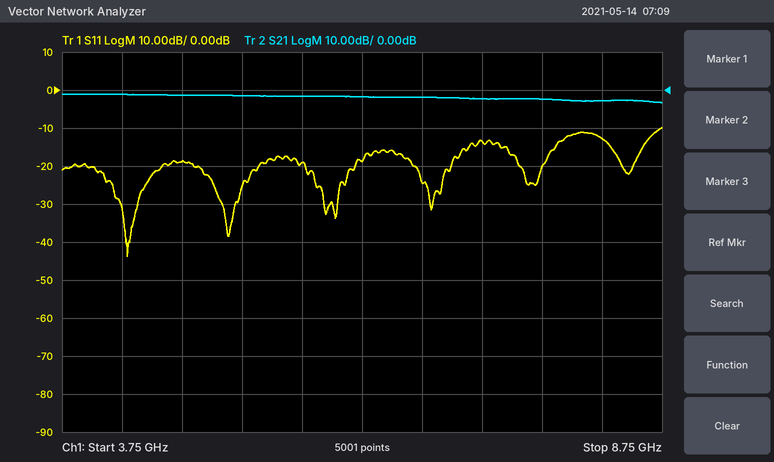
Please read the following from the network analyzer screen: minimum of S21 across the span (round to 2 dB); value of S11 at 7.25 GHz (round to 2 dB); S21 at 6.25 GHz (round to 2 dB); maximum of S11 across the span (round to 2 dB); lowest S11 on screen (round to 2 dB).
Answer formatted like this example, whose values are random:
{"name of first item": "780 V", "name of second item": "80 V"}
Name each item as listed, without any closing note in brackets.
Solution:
{"minimum of S21 across the span": "-4 dB", "value of S11 at 7.25 GHz": "-14 dB", "S21 at 6.25 GHz": "-2 dB", "maximum of S11 across the span": "-10 dB", "lowest S11 on screen": "-44 dB"}
